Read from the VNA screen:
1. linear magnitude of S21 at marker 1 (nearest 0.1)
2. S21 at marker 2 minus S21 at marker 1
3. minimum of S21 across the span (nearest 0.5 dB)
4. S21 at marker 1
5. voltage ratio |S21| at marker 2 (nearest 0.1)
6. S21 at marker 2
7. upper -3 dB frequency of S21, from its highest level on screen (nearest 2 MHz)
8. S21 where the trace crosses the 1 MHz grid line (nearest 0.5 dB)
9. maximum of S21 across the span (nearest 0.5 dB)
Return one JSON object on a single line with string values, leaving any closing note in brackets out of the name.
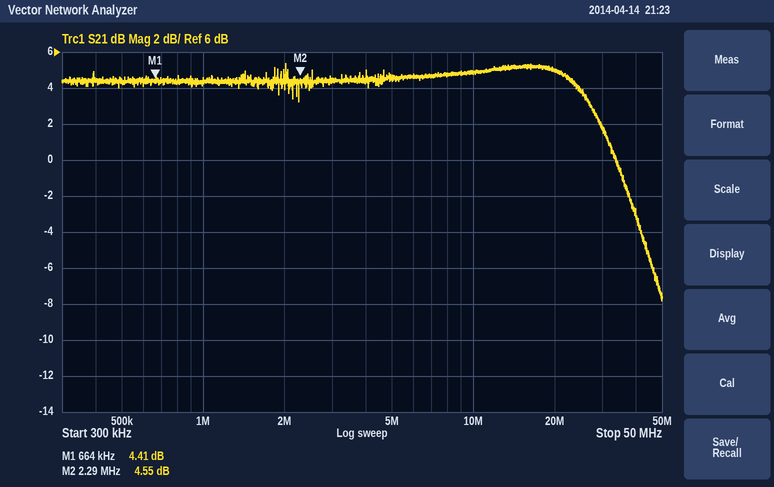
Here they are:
{"linear magnitude of S21 at marker 1": "1.7", "S21 at marker 2 minus S21 at marker 1": "0.14 dB", "minimum of S21 across the span": "-8.0 dB", "S21 at marker 1": "4.41 dB", "voltage ratio |S21| at marker 2": "1.7", "S21 at marker 2": "4.55 dB", "upper -3 dB frequency of S21, from its highest level on screen": "28 MHz", "S21 where the trace crosses the 1 MHz grid line": "4.5 dB", "maximum of S21 across the span": "5.5 dB"}
